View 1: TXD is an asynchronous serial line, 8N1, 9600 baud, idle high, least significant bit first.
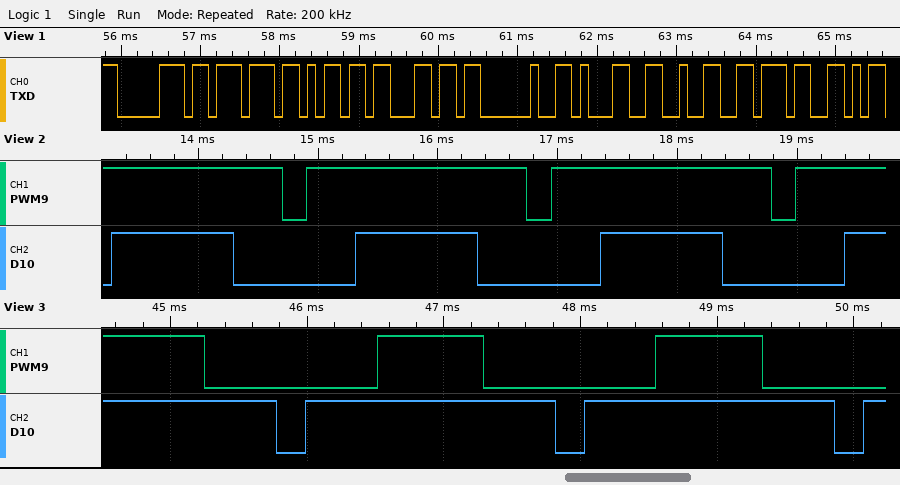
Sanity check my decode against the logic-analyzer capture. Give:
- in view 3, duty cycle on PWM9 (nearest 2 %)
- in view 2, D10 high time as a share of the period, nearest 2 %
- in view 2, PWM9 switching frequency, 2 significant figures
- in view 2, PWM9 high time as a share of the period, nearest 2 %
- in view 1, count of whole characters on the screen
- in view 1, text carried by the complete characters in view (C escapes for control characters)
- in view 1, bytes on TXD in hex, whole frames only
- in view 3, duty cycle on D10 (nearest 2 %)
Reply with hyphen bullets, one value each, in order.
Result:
- 38 %
- 50 %
- 490 Hz
- 90 %
- 8
- "pwml 127"
- 70 77 6D 6C 20 31 32 37
- 90 %
